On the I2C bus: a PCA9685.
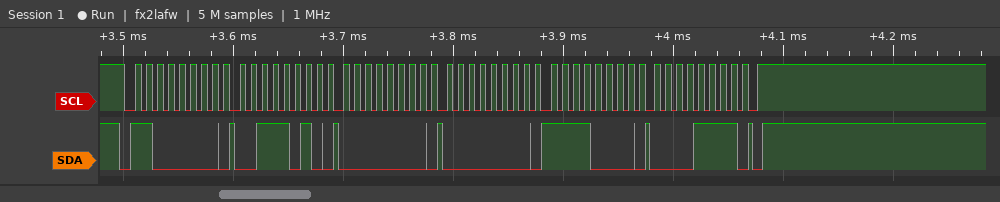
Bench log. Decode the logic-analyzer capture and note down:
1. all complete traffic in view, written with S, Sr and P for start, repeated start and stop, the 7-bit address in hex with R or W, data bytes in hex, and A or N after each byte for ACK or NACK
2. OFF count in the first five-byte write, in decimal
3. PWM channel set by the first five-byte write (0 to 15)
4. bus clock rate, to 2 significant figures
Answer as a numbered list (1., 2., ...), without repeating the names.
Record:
1. S 60W A 3A A 00 A 00 A F0 A 0F A P
2. 4080
3. 13
4. 100 kHz
